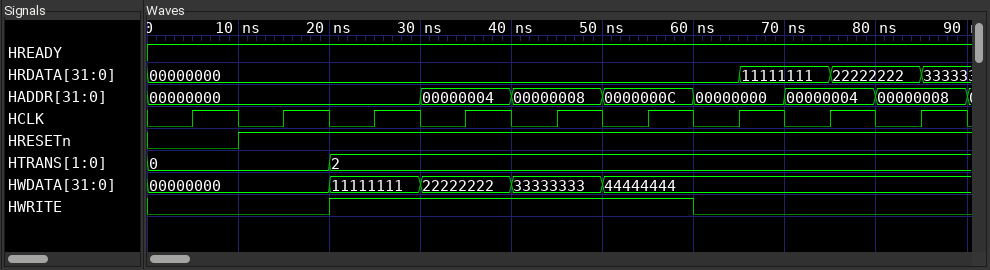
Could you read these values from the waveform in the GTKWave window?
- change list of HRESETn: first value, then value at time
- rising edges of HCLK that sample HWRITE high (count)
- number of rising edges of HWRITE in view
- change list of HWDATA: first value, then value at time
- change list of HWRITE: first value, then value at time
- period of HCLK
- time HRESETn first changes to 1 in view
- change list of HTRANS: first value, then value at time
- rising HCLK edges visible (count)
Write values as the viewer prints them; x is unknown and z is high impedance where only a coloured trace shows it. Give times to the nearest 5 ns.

0, 1 at 10 ns
4
1
00000000, 11111111 at 20 ns, 22222222 at 30 ns, 33333333 at 40 ns, 44444444 at 50 ns
0, 1 at 20 ns, 0 at 60 ns
10 ns
10 ns
0, 2 at 20 ns
9
